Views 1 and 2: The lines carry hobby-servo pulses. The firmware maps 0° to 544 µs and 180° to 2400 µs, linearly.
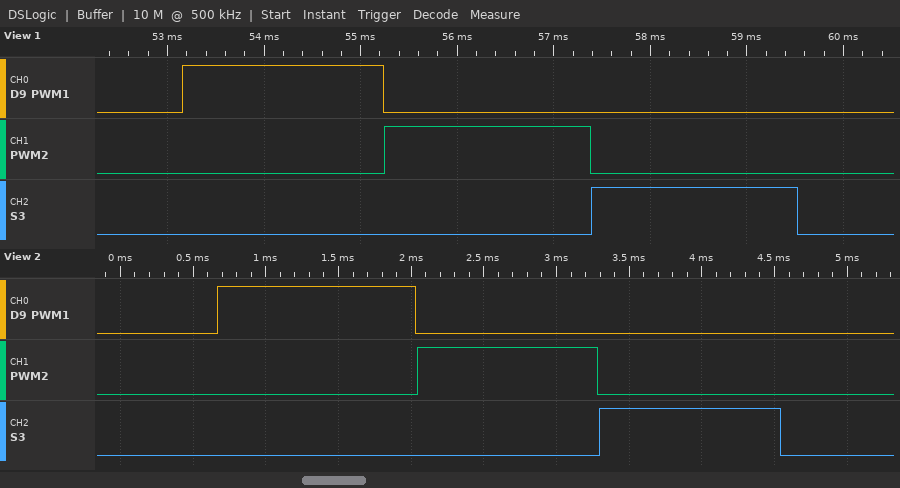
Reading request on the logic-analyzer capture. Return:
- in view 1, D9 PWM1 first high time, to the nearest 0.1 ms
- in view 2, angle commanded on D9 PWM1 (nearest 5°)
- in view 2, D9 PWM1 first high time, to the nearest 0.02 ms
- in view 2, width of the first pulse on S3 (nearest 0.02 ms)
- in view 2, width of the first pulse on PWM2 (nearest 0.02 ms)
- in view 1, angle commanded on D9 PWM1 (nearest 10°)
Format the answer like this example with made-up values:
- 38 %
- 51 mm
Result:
- 2.1 ms
- 80°
- 1.36 ms
- 1.24 ms
- 1.24 ms
- 150°
